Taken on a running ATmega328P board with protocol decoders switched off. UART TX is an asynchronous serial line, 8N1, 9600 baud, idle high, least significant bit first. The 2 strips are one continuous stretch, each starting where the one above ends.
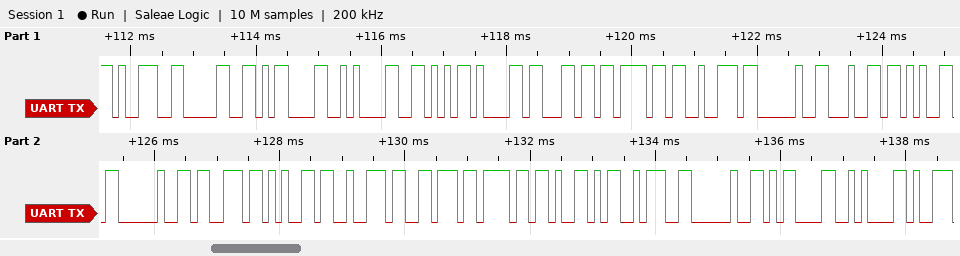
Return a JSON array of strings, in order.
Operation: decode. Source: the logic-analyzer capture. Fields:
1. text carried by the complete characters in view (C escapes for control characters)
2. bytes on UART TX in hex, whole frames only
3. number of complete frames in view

["\"90\\r\\nValor de servoY: \\r\\n\"", "39 30 0D 0A 56 61 6C 6F 72 20 64 65 20 73 65 72 76 6F 59 3A 20 0D 0A", "23"]
